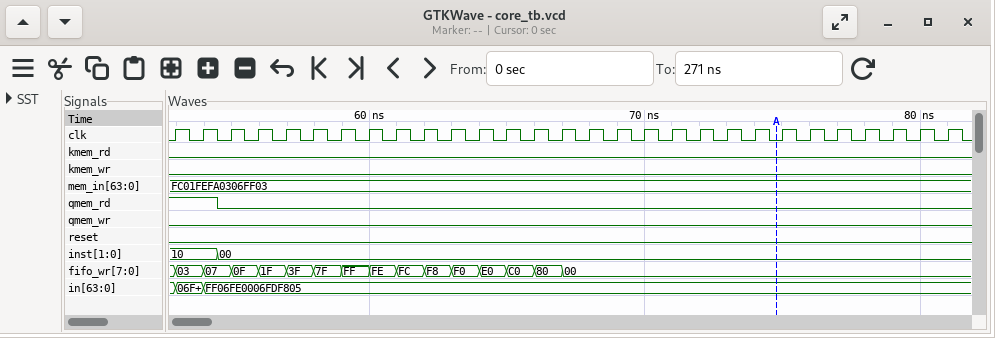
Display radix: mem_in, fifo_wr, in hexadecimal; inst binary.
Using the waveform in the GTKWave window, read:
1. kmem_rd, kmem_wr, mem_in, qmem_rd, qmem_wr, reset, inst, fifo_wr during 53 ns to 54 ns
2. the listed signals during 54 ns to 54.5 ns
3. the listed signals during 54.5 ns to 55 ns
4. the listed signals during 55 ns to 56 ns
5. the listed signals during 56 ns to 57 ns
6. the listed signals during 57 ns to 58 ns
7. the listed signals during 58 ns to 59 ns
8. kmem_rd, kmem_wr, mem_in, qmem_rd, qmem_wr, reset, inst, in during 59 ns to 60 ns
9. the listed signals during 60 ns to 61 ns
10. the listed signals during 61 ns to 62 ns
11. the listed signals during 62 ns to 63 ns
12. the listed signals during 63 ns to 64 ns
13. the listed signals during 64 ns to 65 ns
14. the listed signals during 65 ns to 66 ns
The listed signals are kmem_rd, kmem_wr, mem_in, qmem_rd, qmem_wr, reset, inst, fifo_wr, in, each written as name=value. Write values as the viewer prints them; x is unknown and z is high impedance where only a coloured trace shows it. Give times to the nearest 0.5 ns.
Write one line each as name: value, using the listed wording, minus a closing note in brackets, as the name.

kmem_rd, kmem_wr, mem_in, qmem_rd, qmem_wr, reset, inst, fifo_wr during 53 ns to 54 ns: kmem_rd=0, kmem_wr=0, mem_in=FC01FEFA0306FF03, qmem_rd=1, qmem_wr=0, reset=0, inst=10, fifo_wr=03
the listed signals during 54 ns to 54.5 ns: kmem_rd=0, kmem_wr=0, mem_in=FC01FEFA0306FF03, qmem_rd=1, qmem_wr=0, reset=0, inst=10, fifo_wr=07, in=FF06FE0006FDF805
the listed signals during 54.5 ns to 55 ns: kmem_rd=0, kmem_wr=0, mem_in=FC01FEFA0306FF03, qmem_rd=0, qmem_wr=0, reset=0, inst=00, fifo_wr=07, in=FF06FE0006FDF805
the listed signals during 55 ns to 56 ns: kmem_rd=0, kmem_wr=0, mem_in=FC01FEFA0306FF03, qmem_rd=0, qmem_wr=0, reset=0, inst=00, fifo_wr=0F, in=FF06FE0006FDF805
the listed signals during 56 ns to 57 ns: kmem_rd=0, kmem_wr=0, mem_in=FC01FEFA0306FF03, qmem_rd=0, qmem_wr=0, reset=0, inst=00, fifo_wr=1F, in=FF06FE0006FDF805
the listed signals during 57 ns to 58 ns: kmem_rd=0, kmem_wr=0, mem_in=FC01FEFA0306FF03, qmem_rd=0, qmem_wr=0, reset=0, inst=00, fifo_wr=3F, in=FF06FE0006FDF805
the listed signals during 58 ns to 59 ns: kmem_rd=0, kmem_wr=0, mem_in=FC01FEFA0306FF03, qmem_rd=0, qmem_wr=0, reset=0, inst=00, fifo_wr=7F, in=FF06FE0006FDF805
kmem_rd, kmem_wr, mem_in, qmem_rd, qmem_wr, reset, inst, in during 59 ns to 60 ns: kmem_rd=0, kmem_wr=0, mem_in=FC01FEFA0306FF03, qmem_rd=0, qmem_wr=0, reset=0, inst=00, in=FF06FE0006FDF805
the listed signals during 60 ns to 61 ns: kmem_rd=0, kmem_wr=0, mem_in=FC01FEFA0306FF03, qmem_rd=0, qmem_wr=0, reset=0, inst=00, fifo_wr=FE, in=FF06FE0006FDF805
the listed signals during 61 ns to 62 ns: kmem_rd=0, kmem_wr=0, mem_in=FC01FEFA0306FF03, qmem_rd=0, qmem_wr=0, reset=0, inst=00, fifo_wr=FC, in=FF06FE0006FDF805
the listed signals during 62 ns to 63 ns: kmem_rd=0, kmem_wr=0, mem_in=FC01FEFA0306FF03, qmem_rd=0, qmem_wr=0, reset=0, inst=00, fifo_wr=F8, in=FF06FE0006FDF805
the listed signals during 63 ns to 64 ns: kmem_rd=0, kmem_wr=0, mem_in=FC01FEFA0306FF03, qmem_rd=0, qmem_wr=0, reset=0, inst=00, fifo_wr=F0, in=FF06FE0006FDF805
the listed signals during 64 ns to 65 ns: kmem_rd=0, kmem_wr=0, mem_in=FC01FEFA0306FF03, qmem_rd=0, qmem_wr=0, reset=0, inst=00, fifo_wr=E0, in=FF06FE0006FDF805
the listed signals during 65 ns to 66 ns: kmem_rd=0, kmem_wr=0, mem_in=FC01FEFA0306FF03, qmem_rd=0, qmem_wr=0, reset=0, inst=00, fifo_wr=C0, in=FF06FE0006FDF805
